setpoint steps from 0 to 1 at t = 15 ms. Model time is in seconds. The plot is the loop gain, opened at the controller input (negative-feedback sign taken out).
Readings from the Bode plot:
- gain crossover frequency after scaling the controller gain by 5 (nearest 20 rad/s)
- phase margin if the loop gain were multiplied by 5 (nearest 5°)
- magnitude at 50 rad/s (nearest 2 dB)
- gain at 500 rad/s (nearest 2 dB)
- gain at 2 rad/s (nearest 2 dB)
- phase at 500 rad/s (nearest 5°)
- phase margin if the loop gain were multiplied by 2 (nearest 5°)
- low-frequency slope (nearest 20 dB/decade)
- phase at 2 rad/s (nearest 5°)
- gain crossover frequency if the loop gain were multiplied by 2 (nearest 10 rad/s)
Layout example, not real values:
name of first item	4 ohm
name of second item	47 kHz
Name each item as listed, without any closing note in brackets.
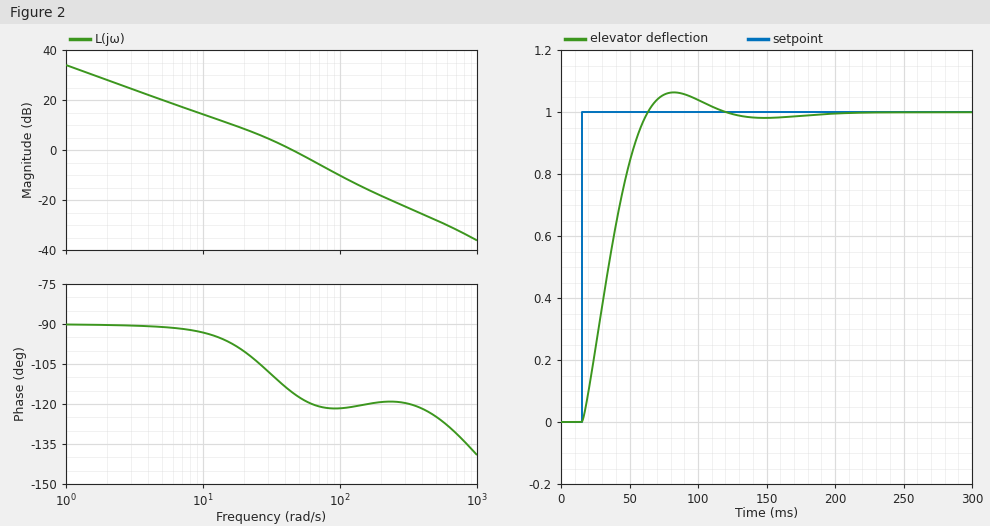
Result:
gain crossover frequency after scaling the controller gain by 5	140 rad/s
phase margin if the loop gain were multiplied by 5	60°
magnitude at 50 rad/s	-2 dB
gain at 500 rad/s	-28 dB
gain at 2 rad/s	28 dB
phase at 500 rad/s	-125°
phase margin if the loop gain were multiplied by 2	60°
low-frequency slope	-20 dB/decade
phase at 2 rad/s	-90°
gain crossover frequency if the loop gain were multiplied by 2	70 rad/s
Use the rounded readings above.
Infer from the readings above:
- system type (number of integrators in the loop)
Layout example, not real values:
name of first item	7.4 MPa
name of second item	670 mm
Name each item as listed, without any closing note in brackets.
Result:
system type	1
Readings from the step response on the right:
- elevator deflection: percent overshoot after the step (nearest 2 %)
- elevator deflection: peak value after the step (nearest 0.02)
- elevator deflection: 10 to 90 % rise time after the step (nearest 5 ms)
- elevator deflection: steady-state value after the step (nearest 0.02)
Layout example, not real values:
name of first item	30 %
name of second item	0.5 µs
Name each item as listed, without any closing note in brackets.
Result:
elevator deflection: percent overshoot after the step	6 %
elevator deflection: peak value after the step	1.06
elevator deflection: 10 to 90 % rise time after the step	35 ms
elevator deflection: steady-state value after the step	1.00
